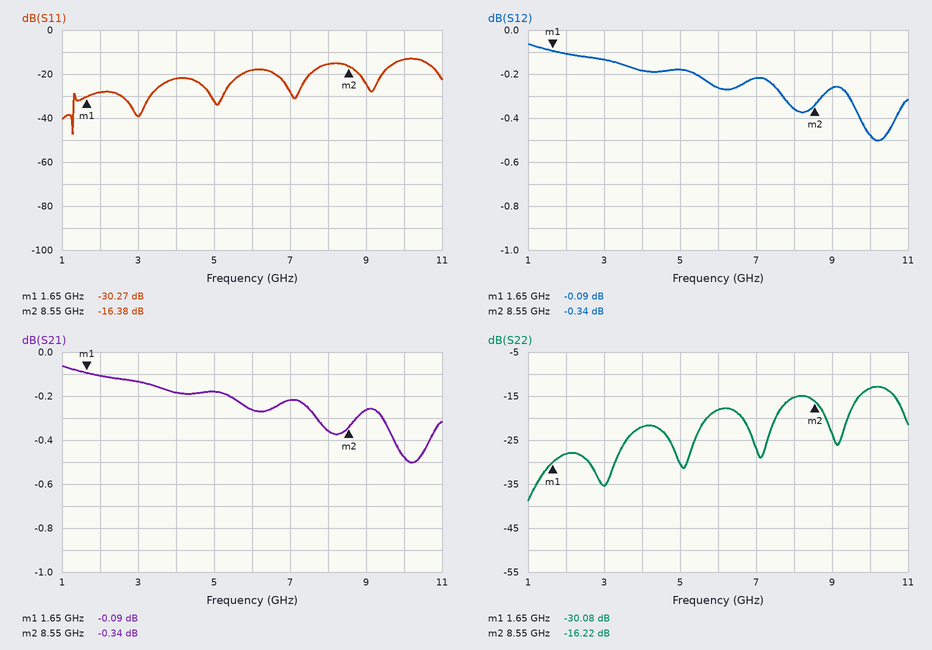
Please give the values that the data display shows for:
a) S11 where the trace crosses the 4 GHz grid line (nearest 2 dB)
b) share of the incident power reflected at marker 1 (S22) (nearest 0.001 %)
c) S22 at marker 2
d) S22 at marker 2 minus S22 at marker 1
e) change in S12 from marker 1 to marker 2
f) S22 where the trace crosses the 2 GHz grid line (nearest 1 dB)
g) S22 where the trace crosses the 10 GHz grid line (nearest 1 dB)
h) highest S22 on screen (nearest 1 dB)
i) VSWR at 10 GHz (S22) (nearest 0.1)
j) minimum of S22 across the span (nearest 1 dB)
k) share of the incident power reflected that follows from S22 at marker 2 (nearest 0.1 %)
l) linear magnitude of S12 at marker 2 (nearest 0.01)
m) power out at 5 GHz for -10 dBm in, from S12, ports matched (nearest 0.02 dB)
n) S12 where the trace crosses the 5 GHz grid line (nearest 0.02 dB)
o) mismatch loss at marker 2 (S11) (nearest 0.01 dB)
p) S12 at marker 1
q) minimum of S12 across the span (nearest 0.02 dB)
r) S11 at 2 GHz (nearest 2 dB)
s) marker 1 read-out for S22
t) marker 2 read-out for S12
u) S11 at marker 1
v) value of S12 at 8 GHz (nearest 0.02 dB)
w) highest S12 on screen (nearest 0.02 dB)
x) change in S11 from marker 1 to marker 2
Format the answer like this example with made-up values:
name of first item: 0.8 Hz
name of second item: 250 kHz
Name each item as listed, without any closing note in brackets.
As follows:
S11 where the trace crosses the 4 GHz grid line: -22 dB
share of the incident power reflected at marker 1 (S22): 0.098 %
S22 at marker 2: -16.22 dB
S22 at marker 2 minus S22 at marker 1: 13.86 dB
change in S12 from marker 1 to marker 2: -0.25 dB
S22 where the trace crosses the 2 GHz grid line: -28 dB
S22 where the trace crosses the 10 GHz grid line: -13 dB
highest S22 on screen: -13 dB
VSWR at 10 GHz (S22): 1.6
minimum of S22 across the span: -39 dB
share of the incident power reflected that follows from S22 at marker 2: 2.4 %
linear magnitude of S12 at marker 2: 0.96
power out at 5 GHz for -10 dBm in, from S12, ports matched: -10.18 dBm
S12 where the trace crosses the 5 GHz grid line: -0.18 dB
mismatch loss at marker 2 (S11): 0.10 dB
S12 at marker 1: -0.09 dB
minimum of S12 across the span: -0.50 dB
S11 at 2 GHz: -28 dB
marker 1 read-out for S22: -30.08 dB
marker 2 read-out for S12: -0.34 dB
S11 at marker 1: -30.27 dB
value of S12 at 8 GHz: -0.36 dB
highest S12 on screen: -0.06 dB
change in S11 from marker 1 to marker 2: 13.89 dB
